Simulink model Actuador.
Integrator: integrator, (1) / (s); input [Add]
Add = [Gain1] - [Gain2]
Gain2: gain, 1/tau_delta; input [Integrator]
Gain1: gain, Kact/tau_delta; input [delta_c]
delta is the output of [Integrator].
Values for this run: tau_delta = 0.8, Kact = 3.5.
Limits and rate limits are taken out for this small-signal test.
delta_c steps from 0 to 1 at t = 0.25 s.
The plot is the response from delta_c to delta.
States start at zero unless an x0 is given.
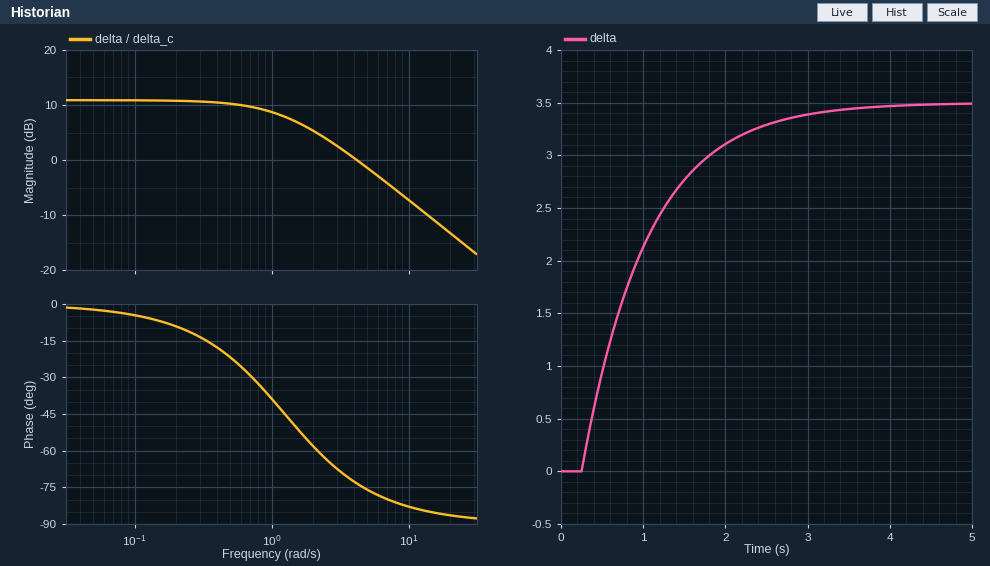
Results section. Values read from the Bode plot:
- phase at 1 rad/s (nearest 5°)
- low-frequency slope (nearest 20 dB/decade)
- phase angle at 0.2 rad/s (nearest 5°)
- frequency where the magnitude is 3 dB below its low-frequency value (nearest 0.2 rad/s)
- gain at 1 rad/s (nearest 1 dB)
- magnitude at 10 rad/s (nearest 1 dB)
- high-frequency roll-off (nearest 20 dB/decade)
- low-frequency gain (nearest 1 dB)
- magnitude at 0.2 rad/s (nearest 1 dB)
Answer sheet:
-40°
0 dB/decade
-10°
1.2 rad/s
9 dB
-7 dB
-20 dB/decade
11 dB
11 dB
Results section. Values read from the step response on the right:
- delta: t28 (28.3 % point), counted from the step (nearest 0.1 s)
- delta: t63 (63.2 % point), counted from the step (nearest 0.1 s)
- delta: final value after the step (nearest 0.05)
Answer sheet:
0.3 s
0.8 s
3.50
